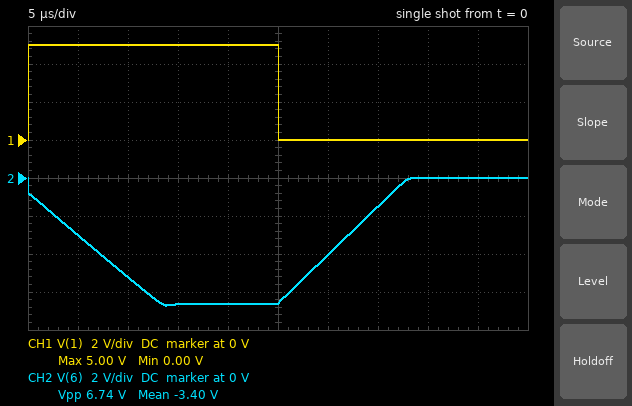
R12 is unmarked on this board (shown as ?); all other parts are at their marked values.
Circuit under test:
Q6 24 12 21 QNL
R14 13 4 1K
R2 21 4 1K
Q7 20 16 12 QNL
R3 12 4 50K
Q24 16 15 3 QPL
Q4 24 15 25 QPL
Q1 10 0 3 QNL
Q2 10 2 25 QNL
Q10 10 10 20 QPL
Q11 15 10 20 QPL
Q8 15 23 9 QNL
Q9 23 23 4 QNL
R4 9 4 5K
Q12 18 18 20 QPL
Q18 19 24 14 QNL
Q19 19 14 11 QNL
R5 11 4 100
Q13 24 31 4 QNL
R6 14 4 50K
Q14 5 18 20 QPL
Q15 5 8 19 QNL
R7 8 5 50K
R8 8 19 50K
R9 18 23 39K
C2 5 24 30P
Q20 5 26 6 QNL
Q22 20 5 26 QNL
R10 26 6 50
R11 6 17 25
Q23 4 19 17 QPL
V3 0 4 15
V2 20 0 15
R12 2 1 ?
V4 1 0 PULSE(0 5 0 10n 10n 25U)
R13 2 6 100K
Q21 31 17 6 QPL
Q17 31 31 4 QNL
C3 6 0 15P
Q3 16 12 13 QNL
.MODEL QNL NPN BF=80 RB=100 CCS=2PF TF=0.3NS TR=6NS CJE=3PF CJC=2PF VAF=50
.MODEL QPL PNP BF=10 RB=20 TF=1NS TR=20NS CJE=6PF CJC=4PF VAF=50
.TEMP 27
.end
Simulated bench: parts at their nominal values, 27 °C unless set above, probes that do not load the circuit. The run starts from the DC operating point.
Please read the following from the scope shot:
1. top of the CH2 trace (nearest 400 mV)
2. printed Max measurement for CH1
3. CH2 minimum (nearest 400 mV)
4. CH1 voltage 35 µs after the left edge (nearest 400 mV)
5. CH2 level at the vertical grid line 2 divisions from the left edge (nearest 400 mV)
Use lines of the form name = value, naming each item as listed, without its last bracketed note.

top of the CH2 trace = 0 V
printed Max measurement for CH1 = 5.00 V
CH2 minimum = -6.8 V
CH1 voltage 35 µs after the left edge = 0 V
CH2 level at the vertical grid line 2 divisions from the left edge = -5.2 V
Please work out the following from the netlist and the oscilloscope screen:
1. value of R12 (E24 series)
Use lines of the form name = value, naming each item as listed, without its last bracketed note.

value of R12 = 75 kΩ
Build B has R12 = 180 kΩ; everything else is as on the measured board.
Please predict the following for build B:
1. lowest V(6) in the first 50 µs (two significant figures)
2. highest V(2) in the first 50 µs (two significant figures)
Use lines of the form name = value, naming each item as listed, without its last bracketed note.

lowest V(6) in the first 50 µs = -2.8 V
highest V(2) in the first 50 µs = 1.5 V
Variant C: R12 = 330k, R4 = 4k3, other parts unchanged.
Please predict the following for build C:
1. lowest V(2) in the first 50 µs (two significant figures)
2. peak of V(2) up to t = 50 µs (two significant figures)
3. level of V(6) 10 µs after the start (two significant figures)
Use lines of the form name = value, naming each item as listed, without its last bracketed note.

lowest V(2) in the first 50 µs = -880 mV
peak of V(2) up to t = 50 µs = 970 mV
level of V(6) 10 µs after the start = -1.5 V
